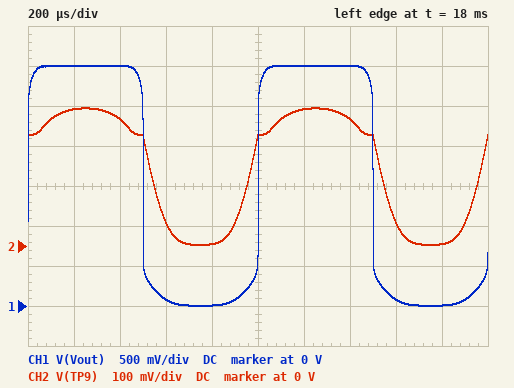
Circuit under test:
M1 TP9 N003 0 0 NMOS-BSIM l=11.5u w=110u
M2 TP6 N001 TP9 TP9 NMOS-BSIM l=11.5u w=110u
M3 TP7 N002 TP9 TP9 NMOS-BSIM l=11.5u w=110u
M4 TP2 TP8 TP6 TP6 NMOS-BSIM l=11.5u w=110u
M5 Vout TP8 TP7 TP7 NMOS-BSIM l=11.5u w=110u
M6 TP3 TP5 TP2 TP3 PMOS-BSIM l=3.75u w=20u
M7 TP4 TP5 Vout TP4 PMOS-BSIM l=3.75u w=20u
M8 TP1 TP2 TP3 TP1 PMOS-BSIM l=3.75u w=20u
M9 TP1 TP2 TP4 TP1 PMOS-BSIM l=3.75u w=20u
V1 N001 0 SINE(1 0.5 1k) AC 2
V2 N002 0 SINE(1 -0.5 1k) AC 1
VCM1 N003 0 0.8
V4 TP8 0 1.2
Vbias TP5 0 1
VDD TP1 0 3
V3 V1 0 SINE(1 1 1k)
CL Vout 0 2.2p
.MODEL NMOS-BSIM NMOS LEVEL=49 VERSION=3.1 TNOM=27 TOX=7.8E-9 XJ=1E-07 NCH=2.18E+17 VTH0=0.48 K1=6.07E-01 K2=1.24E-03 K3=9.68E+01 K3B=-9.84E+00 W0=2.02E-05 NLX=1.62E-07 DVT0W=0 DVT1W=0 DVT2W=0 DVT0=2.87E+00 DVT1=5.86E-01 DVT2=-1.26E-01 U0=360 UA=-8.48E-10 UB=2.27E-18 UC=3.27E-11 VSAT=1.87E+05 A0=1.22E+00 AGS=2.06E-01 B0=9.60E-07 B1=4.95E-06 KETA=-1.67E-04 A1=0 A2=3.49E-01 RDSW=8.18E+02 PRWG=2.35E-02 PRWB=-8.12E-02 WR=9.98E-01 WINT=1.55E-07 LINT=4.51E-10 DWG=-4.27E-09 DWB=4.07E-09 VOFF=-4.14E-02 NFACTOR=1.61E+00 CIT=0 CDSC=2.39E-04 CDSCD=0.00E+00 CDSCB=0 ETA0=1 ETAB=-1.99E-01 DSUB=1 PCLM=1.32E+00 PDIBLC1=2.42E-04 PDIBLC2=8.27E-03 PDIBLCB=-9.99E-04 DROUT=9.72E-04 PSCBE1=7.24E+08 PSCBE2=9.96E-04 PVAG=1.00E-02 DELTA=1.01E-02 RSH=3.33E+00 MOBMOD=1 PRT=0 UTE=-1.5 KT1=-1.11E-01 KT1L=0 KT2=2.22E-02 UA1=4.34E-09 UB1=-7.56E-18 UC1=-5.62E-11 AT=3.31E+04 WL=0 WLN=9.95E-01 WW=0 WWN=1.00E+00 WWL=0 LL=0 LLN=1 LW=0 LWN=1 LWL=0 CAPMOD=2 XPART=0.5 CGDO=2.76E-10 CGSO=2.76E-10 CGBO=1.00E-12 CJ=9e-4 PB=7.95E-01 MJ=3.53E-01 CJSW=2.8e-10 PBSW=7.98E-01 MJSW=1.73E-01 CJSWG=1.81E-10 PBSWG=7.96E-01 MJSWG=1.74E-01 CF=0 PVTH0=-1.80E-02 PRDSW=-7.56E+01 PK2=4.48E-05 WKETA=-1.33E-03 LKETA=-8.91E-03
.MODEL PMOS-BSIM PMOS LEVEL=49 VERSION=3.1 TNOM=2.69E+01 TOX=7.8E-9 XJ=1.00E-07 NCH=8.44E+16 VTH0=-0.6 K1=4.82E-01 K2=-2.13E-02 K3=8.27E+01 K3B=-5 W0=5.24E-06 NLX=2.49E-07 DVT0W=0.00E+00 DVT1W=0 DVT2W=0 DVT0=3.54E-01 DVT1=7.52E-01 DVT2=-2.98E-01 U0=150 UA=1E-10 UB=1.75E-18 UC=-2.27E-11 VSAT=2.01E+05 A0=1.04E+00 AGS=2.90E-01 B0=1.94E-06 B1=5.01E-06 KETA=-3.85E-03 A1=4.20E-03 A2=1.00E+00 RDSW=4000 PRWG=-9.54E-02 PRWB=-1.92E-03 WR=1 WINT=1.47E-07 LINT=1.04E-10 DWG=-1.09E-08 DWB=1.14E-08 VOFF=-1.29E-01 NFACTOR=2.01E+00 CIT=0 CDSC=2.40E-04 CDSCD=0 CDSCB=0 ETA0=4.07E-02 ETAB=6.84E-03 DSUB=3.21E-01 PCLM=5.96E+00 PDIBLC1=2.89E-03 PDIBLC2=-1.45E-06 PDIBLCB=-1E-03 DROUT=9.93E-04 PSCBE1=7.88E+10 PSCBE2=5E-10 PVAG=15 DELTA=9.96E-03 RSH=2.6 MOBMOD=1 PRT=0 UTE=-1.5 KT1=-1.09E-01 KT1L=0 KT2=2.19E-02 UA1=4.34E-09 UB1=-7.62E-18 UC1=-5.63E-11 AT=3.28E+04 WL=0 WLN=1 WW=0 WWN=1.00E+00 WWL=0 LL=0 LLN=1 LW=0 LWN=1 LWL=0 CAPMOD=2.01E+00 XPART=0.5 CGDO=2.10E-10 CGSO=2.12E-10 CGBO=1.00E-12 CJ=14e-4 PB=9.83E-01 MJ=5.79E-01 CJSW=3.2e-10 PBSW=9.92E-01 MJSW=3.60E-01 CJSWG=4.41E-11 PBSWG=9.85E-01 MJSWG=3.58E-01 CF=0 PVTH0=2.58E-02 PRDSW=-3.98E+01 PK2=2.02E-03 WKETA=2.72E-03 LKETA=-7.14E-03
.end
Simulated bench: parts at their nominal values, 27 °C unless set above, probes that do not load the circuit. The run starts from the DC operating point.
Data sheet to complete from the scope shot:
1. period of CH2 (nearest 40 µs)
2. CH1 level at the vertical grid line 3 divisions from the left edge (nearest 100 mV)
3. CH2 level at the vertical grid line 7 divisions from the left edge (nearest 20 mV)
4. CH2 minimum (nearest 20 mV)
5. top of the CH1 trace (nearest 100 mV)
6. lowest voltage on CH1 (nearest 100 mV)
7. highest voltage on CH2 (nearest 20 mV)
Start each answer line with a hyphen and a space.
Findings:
- 1.00 ms
- 100 mV
- 320 mV
- 0 V
- 3.0 V
- 0 V
- 340 mV
